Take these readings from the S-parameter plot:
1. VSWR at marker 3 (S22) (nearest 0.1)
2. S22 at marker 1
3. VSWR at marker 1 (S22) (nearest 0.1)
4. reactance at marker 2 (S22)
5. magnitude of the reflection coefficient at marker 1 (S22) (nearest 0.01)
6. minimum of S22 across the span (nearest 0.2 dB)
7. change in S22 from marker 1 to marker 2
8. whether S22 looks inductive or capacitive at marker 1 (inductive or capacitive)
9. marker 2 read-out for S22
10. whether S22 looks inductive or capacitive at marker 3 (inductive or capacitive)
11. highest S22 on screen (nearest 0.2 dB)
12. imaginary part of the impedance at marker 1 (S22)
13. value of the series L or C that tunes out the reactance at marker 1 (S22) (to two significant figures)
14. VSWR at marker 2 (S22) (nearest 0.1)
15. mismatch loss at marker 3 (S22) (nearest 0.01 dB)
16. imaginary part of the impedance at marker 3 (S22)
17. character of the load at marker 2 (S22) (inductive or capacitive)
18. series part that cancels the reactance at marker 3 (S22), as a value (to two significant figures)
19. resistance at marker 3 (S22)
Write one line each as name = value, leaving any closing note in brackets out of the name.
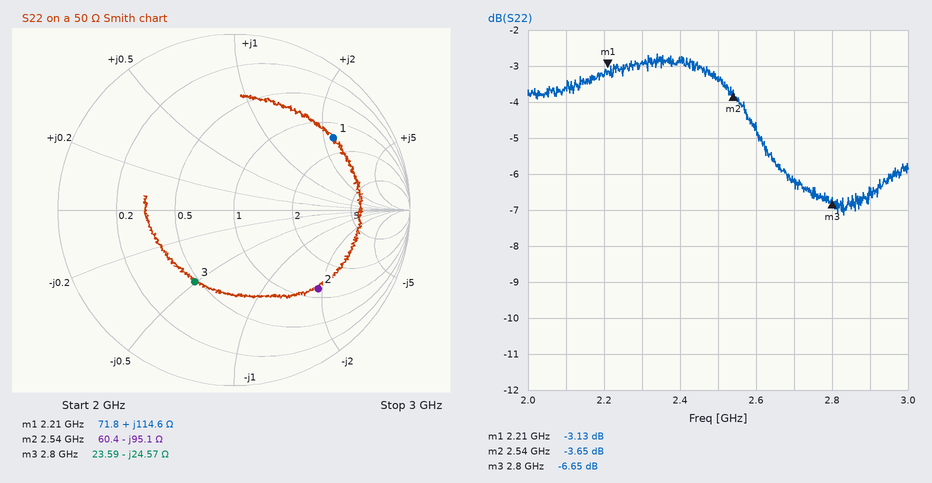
VSWR at marker 3 (S22) = 2.7
S22 at marker 1 = -3.13 dB
VSWR at marker 1 (S22) = 5.6
reactance at marker 2 = -95.1 Ω
magnitude of the reflection coefficient at marker 1 (S22) = 0.70
minimum of S22 across the span = -7.2 dB
change in S22 from marker 1 to marker 2 = -0.52 dB
whether S22 looks inductive or capacitive at marker 1 = inductive
marker 2 read-out for S22 = -3.65 dB
whether S22 looks inductive or capacitive at marker 3 = capacitive
highest S22 on screen = -2.6 dB
imaginary part of the impedance at marker 1 = +114.6 Ω
value of the series L or C that tunes out the reactance at marker 1 (S22) = 630 fF
VSWR at marker 2 (S22) = 4.8
mismatch loss at marker 3 (S22) = 1.06 dB
imaginary part of the impedance at marker 3 = -24.57 Ω
character of the load at marker 2 (S22) = capacitive
series part that cancels the reactance at marker 3 (S22), as a value = 1.4 nH
resistance at marker 3 = 23.59 Ω
